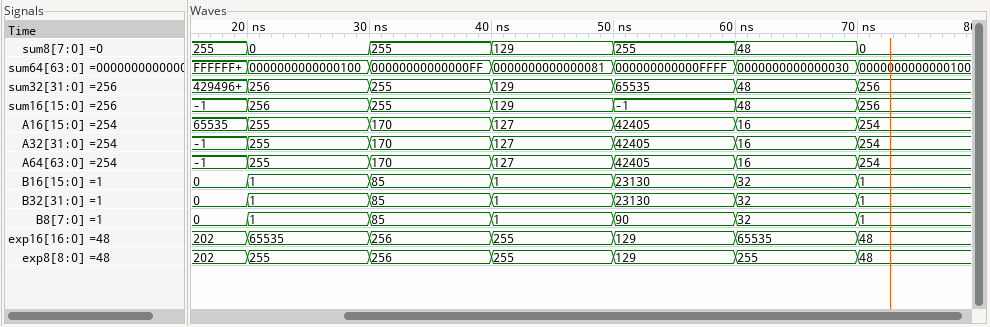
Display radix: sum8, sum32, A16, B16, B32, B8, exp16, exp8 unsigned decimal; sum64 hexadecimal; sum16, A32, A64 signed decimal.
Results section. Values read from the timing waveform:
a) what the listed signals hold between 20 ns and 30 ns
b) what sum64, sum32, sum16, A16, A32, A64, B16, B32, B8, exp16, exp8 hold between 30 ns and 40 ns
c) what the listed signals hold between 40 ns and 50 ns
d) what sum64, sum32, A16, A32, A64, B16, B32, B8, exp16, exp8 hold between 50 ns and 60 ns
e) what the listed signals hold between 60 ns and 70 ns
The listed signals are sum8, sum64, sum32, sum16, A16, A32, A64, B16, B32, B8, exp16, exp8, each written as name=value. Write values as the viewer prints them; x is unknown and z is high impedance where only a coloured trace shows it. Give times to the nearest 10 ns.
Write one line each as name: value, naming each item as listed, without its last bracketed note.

what the listed signals hold between 20 ns and 30 ns: sum8=0, sum64=0000000000000100, sum32=256, sum16=256, A16=255, A32=255, A64=255, B16=1, B32=1, B8=1, exp16=65535, exp8=255
what sum64, sum32, sum16, A16, A32, A64, B16, B32, B8, exp16, exp8 hold between 30 ns and 40 ns: sum64=00000000000000FF, sum32=255, sum16=255, A16=170, A32=170, A64=170, B16=85, B32=85, B8=85, exp16=256, exp8=256
what the listed signals hold between 40 ns and 50 ns: sum8=129, sum64=0000000000000081, sum32=129, sum16=129, A16=127, A32=127, A64=127, B16=1, B32=1, B8=1, exp16=255, exp8=255
what sum64, sum32, A16, A32, A64, B16, B32, B8, exp16, exp8 hold between 50 ns and 60 ns: sum64=000000000000FFFF, sum32=65535, A16=42405, A32=42405, A64=42405, B16=23130, B32=23130, B8=90, exp16=129, exp8=129
what the listed signals hold between 60 ns and 70 ns: sum8=48, sum64=0000000000000030, sum32=48, sum16=48, A16=16, A32=16, A64=16, B16=32, B32=32, B8=32, exp16=65535, exp8=255
